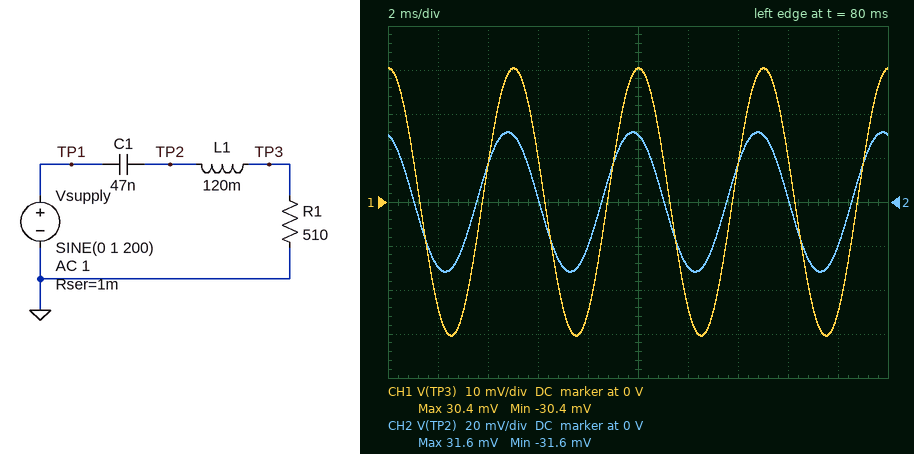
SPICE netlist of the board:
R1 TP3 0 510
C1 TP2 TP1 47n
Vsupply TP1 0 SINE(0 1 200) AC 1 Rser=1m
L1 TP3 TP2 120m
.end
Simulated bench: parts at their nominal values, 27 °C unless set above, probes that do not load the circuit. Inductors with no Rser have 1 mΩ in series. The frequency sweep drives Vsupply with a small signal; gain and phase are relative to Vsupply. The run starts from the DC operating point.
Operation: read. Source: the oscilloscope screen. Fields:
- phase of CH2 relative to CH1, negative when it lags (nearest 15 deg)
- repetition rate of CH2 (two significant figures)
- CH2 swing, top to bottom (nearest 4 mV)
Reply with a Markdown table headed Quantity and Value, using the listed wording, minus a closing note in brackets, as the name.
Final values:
| Quantity | Value |
|---|---|
| phase of CH2 relative to CH1, negative when it lags | 15 deg |
| repetition rate of CH2 | 200 Hz |
| CH2 swing, top to bottom | 64 mV |
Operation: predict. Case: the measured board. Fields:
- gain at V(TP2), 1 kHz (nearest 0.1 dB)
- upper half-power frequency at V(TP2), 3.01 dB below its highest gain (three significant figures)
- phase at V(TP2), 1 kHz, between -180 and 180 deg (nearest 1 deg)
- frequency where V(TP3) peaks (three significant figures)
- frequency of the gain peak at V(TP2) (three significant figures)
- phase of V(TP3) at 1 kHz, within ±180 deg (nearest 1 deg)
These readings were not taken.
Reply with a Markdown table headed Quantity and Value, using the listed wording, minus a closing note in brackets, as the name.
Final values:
| Quantity | Value |
|---|---|
| gain at V(TP2), 1 kHz | -9.4 dB |
| upper half-power frequency at V(TP2), 3.01 dB below its highest gain | 2.64 kHz |
| phase at V(TP2), 1 kHz, between -180 and 180 deg | 135 deg |
| frequency where V(TP3) peaks | 2.12 kHz |
| frequency of the gain peak at V(TP2) | 2.17 kHz |
| phase of V(TP3) at 1 kHz, within ±180 deg | 79 deg |
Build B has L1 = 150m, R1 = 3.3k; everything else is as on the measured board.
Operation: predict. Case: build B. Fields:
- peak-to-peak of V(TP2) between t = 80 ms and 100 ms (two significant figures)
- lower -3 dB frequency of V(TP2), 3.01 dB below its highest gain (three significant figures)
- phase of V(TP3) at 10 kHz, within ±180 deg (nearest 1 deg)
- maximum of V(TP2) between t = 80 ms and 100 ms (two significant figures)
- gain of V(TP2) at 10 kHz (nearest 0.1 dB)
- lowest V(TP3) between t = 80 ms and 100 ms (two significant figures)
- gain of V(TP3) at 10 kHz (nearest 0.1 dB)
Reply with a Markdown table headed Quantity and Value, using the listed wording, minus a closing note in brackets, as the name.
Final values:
| Quantity | Value |
|---|---|
| peak-to-peak of V(TP2) between t = 80 ms and 100 ms | 390 mV |
| lower -3 dB frequency of V(TP2), 3.01 dB below its highest gain | 993 Hz |
| phase of V(TP3) at 10 kHz, within ±180 deg | -70 deg |
| maximum of V(TP2) between t = 80 ms and 100 ms | 190 mV |
| gain of V(TP2) at 10 kHz | 0.3 dB |
| lowest V(TP3) between t = 80 ms and 100 ms | -190 mV |
| gain of V(TP3) at 10 kHz | -9.3 dB |
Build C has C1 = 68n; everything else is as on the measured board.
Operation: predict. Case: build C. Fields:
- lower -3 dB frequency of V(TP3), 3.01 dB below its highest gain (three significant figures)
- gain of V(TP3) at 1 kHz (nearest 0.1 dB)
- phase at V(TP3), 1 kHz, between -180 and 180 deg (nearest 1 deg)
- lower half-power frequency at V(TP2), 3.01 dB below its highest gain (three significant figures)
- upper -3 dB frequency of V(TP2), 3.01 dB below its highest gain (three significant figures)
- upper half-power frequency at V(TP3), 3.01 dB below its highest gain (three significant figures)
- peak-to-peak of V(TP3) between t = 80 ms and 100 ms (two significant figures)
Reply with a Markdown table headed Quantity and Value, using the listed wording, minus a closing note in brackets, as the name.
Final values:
| Quantity | Value |
|---|---|
| lower -3 dB frequency of V(TP3), 3.01 dB below its highest gain | 1.46 kHz |
| gain of V(TP3) at 1 kHz | -10.3 dB |
| phase at V(TP3), 1 kHz, between -180 and 180 deg | 72 deg |
| lower half-power frequency at V(TP2), 3.01 dB below its highest gain | 1.53 kHz |
| upper -3 dB frequency of V(TP2), 3.01 dB below its highest gain | 2.34 kHz |
| upper half-power frequency at V(TP3), 3.01 dB below its highest gain | 2.13 kHz |
| peak-to-peak of V(TP3) between t = 80 ms and 100 ms | 88 mV |
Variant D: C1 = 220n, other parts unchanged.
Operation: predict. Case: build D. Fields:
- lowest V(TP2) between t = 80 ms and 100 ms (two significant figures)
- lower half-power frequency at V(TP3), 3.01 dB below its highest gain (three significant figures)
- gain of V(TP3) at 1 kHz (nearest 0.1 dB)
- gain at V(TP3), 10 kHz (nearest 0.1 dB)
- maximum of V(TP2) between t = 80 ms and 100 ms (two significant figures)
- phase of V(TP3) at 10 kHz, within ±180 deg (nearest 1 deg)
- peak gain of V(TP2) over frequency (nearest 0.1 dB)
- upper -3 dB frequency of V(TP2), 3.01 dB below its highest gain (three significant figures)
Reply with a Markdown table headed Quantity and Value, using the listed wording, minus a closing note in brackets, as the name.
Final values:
| Quantity | Value |
|---|---|
| lowest V(TP2) between t = 80 ms and 100 ms | -150 mV |
| lower half-power frequency at V(TP3), 3.01 dB below its highest gain | 698 Hz |
| gain of V(TP3) at 1 kHz | 0 dB |
| gain at V(TP3), 10 kHz | -23.3 dB |
| maximum of V(TP2) between t = 80 ms and 100 ms | 150 mV |
| phase of V(TP3) at 10 kHz, within ±180 deg | -86 deg |
| peak gain of V(TP2) over frequency | 5.2 dB |
| upper -3 dB frequency of V(TP2), 3.01 dB below its highest gain | 1.96 kHz |
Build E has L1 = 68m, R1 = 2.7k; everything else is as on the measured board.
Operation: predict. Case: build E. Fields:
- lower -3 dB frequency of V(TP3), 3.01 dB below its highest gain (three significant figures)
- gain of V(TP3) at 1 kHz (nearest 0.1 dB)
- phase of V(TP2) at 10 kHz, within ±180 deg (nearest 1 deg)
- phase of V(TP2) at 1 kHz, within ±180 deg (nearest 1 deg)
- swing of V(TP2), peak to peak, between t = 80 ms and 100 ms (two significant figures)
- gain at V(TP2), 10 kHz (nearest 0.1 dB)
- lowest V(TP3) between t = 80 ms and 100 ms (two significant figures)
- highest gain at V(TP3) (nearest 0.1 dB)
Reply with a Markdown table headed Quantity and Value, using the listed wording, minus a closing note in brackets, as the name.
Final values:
| Quantity | Value |
|---|---|
| lower -3 dB frequency of V(TP3), 3.01 dB below its highest gain | 1.07 kHz |
| gain of V(TP3) at 1 kHz | -3.4 dB |
| phase of V(TP2) at 10 kHz, within ±180 deg | 2 deg |
| phase of V(TP2) at 1 kHz, within ±180 deg | 57 deg |
| swing of V(TP2), peak to peak, between t = 80 ms and 100 ms | 320 mV |
| gain at V(TP2), 10 kHz | 0.5 dB |
| lowest V(TP3) between t = 80 ms and 100 ms | -160 mV |
| highest gain at V(TP3) | 0 dB |
